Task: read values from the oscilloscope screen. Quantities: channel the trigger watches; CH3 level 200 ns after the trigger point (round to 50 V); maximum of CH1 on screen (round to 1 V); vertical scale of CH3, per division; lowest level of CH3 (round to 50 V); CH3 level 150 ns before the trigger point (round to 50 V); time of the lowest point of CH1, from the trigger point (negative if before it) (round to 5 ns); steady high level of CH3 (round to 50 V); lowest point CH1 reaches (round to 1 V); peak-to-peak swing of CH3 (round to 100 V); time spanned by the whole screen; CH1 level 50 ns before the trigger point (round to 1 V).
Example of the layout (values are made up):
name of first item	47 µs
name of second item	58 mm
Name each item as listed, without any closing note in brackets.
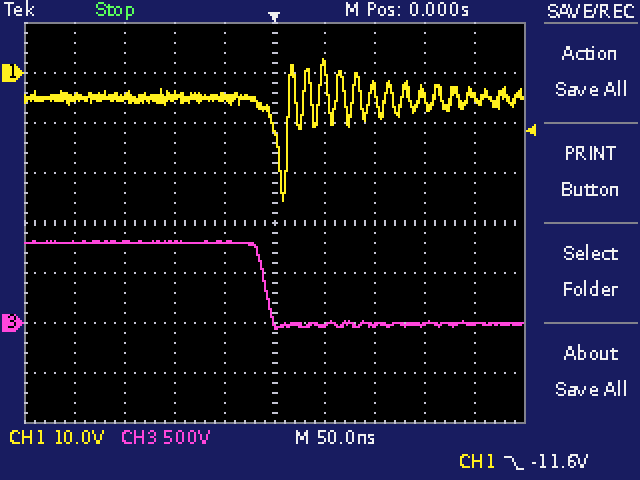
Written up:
channel the trigger watches	CH1
CH3 level 200 ns after the trigger point	0 V
maximum of CH1 on screen	3 V
vertical scale of CH3, per division	500 V
lowest level of CH3	-50 V
CH3 level 150 ns before the trigger point	800 V
time of the lowest point of CH1, from the trigger point (negative if before it)	+10 ns
steady high level of CH3	800 V
lowest point CH1 reaches	-26 V
peak-to-peak swing of CH3	900 V
time spanned by the whole screen	500 ns
CH1 level 50 ns before the trigger point	-5 V
